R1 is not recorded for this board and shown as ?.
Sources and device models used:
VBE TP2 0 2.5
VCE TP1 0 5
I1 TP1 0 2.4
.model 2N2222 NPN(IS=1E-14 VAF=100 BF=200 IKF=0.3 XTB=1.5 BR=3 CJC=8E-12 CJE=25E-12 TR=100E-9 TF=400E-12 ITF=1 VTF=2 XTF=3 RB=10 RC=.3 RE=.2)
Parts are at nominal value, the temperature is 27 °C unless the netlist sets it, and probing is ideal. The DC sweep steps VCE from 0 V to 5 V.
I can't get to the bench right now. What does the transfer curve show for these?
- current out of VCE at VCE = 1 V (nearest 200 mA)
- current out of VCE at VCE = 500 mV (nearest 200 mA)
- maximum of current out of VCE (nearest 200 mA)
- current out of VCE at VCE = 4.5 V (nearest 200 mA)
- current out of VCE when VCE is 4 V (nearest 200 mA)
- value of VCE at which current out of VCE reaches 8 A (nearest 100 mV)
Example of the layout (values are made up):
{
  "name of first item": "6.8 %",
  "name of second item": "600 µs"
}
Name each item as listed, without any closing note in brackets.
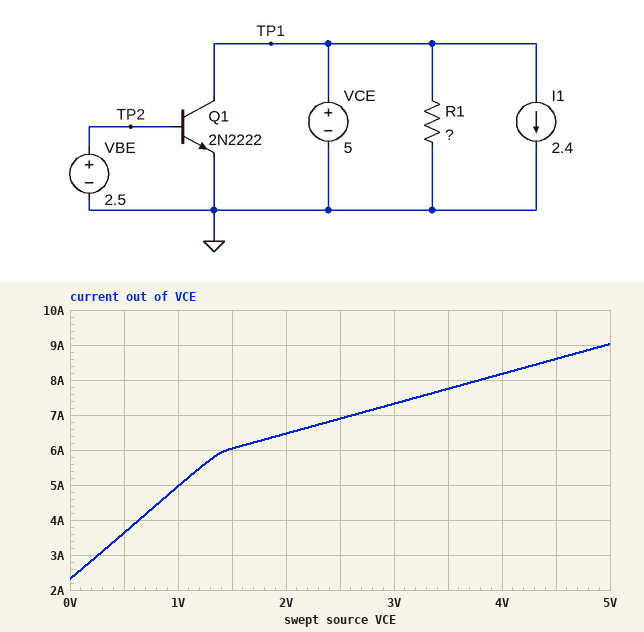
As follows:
{
  "current out of VCE at VCE = 1 V": "5.0 A",
  "current out of VCE at VCE = 500 mV": "3.6 A",
  "maximum of current out of VCE": "9.0 A",
  "current out of VCE at VCE = 4.5 V": "8.6 A",
  "current out of VCE when VCE is 4 V": "8.2 A",
  "value of VCE at which current out of VCE reaches 8 A": "3.8 V"
}
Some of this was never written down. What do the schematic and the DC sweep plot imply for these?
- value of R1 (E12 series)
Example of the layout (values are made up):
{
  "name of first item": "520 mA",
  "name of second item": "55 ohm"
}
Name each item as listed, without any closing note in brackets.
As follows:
{
  "value of R1": "1.2 Ω"
}
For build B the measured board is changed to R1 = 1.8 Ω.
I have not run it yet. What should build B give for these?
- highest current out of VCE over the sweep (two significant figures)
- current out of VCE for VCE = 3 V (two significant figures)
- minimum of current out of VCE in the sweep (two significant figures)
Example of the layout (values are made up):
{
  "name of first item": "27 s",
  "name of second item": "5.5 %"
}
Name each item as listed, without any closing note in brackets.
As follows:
{
  "highest current out of VCE over the sweep": "7.6 A",
  "current out of VCE for VCE = 3 V": "6.5 A",
  "minimum of current out of VCE in the sweep": "2.3 A"
}
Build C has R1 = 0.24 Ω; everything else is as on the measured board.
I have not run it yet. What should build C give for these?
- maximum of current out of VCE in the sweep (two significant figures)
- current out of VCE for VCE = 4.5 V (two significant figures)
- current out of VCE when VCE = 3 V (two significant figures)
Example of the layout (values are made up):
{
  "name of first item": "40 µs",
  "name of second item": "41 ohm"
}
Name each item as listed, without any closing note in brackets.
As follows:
{
  "maximum of current out of VCE in the sweep": "26 A",
  "current out of VCE for VCE = 4.5 V": "24 A",
  "current out of VCE when VCE = 3 V": "17 A"
}
